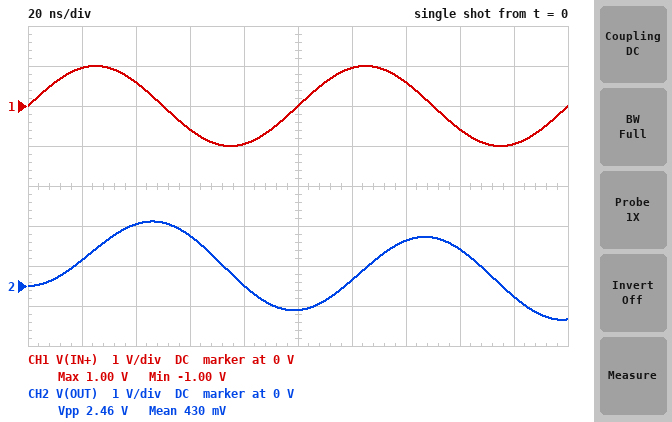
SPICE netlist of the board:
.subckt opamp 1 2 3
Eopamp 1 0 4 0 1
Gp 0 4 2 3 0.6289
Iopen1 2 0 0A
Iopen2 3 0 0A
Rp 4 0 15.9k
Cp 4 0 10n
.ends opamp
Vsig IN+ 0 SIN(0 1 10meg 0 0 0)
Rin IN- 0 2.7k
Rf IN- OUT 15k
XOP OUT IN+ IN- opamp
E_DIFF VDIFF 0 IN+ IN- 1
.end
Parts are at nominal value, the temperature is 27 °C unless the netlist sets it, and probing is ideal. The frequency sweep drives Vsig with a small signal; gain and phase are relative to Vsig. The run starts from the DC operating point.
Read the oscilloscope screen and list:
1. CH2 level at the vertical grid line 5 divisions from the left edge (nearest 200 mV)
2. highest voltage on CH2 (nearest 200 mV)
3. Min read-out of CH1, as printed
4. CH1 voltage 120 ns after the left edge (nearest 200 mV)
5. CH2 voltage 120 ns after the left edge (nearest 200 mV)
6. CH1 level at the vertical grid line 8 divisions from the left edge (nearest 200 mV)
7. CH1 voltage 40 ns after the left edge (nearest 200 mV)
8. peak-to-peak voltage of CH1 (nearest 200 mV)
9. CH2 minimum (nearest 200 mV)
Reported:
-600 mV
1.6 V
-1.00 V
1.0 V
200 mV
-600 mV
600 mV
2.0 V
-800 mV
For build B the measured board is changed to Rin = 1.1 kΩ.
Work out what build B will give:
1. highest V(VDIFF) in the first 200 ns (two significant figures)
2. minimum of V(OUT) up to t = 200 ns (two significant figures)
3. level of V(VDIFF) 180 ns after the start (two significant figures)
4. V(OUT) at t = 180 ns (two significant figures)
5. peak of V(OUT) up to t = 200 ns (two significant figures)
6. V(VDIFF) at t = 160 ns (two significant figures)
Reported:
960 mV
-580 mV
-960 mV
86 mV
1.8 V
-670 mV
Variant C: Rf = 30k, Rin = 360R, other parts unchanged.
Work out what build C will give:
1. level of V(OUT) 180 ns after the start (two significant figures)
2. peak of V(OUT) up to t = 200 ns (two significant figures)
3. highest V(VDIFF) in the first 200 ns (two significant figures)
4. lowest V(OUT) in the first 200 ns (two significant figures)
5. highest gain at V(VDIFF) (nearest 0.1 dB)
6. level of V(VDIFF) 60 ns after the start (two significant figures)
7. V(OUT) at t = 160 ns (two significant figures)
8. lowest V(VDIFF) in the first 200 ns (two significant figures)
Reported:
550 mV
2.0 V
990 mV
-140 mV
0 dB
-610 mV
1.7 V
-1.0 V
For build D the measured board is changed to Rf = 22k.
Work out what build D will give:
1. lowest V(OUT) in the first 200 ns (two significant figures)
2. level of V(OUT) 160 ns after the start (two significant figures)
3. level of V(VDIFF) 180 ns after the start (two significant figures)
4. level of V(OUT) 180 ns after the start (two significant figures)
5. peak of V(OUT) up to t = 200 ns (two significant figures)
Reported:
-740 mV
1.1 V
-940 mV
-120 mV
1.7 V
